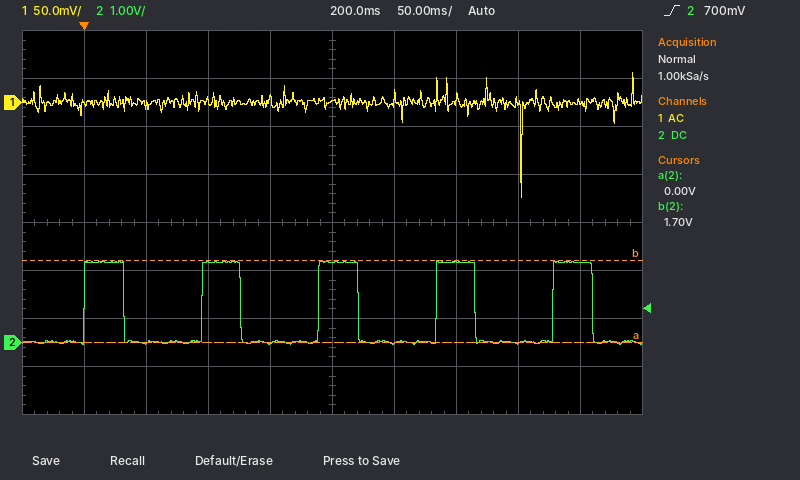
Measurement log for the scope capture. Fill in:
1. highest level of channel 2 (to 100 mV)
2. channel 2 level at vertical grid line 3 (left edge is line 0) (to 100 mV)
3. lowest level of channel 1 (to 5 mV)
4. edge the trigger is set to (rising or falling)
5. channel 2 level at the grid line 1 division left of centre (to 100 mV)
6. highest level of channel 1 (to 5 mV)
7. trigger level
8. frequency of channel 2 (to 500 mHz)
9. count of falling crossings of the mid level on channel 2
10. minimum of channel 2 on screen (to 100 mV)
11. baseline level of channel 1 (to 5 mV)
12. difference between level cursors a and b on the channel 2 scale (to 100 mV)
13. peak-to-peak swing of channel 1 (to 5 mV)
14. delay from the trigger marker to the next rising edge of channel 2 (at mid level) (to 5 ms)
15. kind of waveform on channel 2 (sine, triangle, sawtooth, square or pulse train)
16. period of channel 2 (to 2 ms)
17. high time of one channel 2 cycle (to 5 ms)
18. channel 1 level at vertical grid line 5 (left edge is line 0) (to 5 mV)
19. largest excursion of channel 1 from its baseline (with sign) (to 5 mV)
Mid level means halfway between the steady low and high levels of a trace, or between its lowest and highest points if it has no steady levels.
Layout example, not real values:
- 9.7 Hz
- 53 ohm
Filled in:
- 1.7 V
- 1.7 V
- -100 mV
- rising
- 0.0 V
- 30 mV
- 700 mV
- 10.5 Hz
- 5
- 0.0 V
- 0 mV
- 1.7 V
- 130 mV
- 95 ms
- pulse train
- 94 ms
- 30 ms
- 0 mV
- -100 mV
